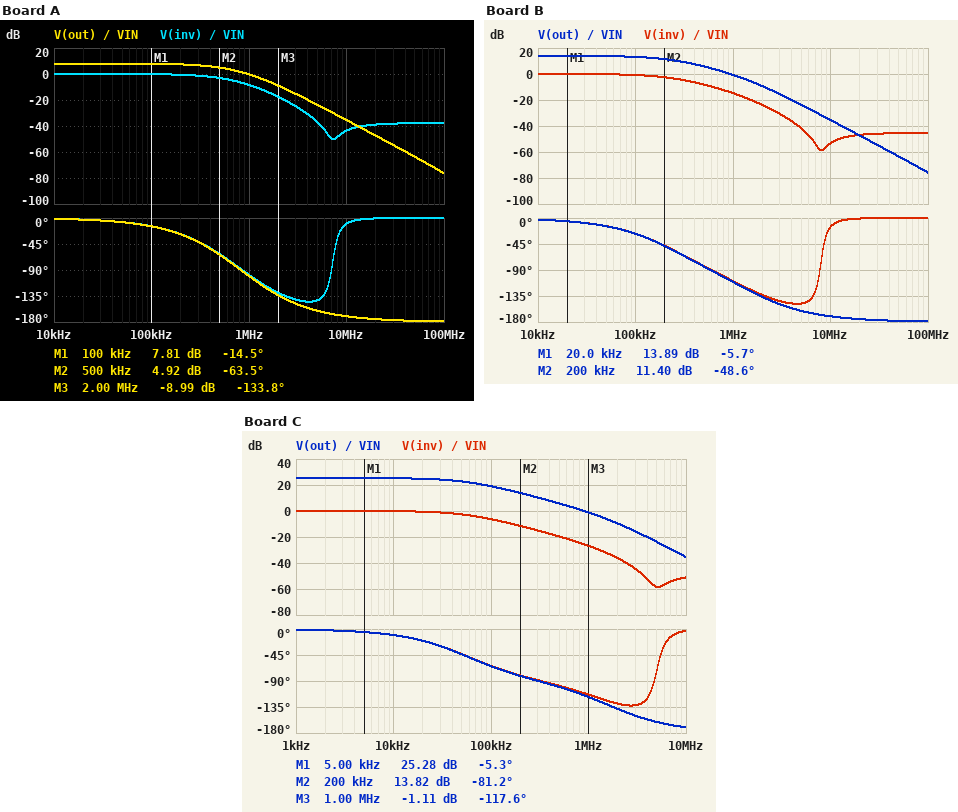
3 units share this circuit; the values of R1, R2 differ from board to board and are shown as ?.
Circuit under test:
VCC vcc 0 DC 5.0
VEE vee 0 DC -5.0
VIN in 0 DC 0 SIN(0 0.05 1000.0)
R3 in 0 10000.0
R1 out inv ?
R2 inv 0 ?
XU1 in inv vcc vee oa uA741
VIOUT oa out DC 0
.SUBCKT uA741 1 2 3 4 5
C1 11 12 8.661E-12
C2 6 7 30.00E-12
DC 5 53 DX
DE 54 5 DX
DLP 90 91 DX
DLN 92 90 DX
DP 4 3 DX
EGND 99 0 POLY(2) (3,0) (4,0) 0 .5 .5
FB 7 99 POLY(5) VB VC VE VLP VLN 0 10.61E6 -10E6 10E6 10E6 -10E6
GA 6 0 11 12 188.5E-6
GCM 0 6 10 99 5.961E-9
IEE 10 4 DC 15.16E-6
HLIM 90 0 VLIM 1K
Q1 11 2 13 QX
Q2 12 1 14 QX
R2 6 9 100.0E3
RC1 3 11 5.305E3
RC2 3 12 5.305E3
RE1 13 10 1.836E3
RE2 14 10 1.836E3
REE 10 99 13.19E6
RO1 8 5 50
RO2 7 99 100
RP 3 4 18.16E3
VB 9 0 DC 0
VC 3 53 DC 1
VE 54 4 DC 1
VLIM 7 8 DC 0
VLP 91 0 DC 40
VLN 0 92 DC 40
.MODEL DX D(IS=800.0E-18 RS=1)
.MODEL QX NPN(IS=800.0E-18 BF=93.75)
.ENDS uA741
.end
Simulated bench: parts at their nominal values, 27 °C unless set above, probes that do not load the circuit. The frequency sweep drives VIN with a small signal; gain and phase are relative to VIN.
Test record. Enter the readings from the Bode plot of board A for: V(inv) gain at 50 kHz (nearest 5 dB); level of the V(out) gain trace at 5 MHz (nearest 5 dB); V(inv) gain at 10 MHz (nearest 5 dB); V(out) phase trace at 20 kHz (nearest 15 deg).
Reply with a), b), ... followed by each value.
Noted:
a) 0 dB
b) -25 dB
c) -45 dB
d) 0 deg
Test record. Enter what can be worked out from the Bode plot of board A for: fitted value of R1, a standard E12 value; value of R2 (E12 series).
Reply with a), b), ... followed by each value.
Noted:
a) 33 kΩ
b) 22 kΩ
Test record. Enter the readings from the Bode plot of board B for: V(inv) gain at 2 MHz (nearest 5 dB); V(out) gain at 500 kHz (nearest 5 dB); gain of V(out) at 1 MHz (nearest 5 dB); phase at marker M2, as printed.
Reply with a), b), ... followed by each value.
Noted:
a) -25 dB
b) 5 dB
c) 0 dB
d) -48.6 deg
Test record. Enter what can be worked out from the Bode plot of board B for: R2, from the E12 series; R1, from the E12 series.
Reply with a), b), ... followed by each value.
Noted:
a) 6.8 kΩ
b) 27 kΩ
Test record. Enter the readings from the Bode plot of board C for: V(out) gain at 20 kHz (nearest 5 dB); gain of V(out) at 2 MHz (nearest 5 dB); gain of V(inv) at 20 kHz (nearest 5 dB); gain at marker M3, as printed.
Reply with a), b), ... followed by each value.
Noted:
a) 25 dB
b) -10 dB
c) 0 dB
d) -1.11 dB
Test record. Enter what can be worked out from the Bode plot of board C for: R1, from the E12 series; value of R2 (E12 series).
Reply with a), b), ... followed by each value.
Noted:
a) 68 kΩ
b) 3.9 kΩ
